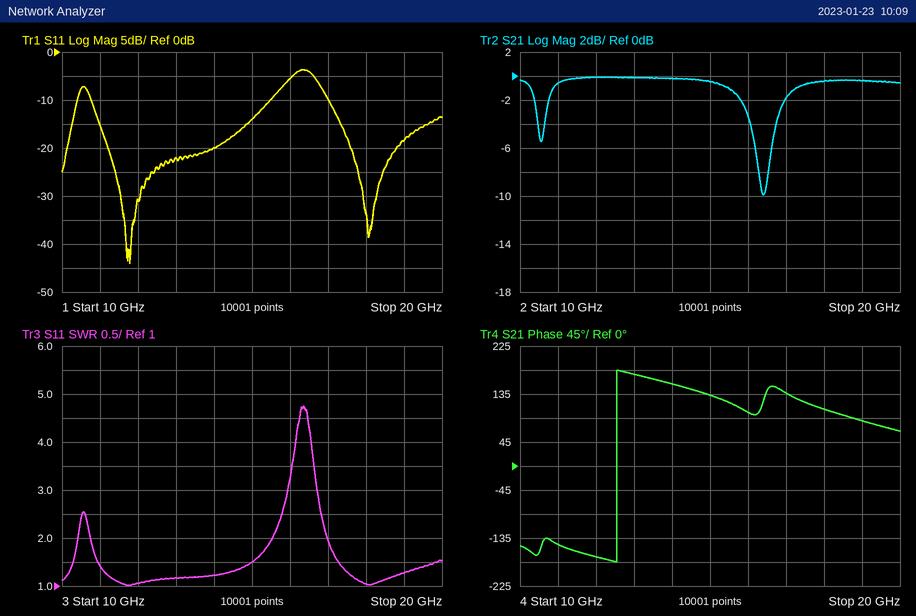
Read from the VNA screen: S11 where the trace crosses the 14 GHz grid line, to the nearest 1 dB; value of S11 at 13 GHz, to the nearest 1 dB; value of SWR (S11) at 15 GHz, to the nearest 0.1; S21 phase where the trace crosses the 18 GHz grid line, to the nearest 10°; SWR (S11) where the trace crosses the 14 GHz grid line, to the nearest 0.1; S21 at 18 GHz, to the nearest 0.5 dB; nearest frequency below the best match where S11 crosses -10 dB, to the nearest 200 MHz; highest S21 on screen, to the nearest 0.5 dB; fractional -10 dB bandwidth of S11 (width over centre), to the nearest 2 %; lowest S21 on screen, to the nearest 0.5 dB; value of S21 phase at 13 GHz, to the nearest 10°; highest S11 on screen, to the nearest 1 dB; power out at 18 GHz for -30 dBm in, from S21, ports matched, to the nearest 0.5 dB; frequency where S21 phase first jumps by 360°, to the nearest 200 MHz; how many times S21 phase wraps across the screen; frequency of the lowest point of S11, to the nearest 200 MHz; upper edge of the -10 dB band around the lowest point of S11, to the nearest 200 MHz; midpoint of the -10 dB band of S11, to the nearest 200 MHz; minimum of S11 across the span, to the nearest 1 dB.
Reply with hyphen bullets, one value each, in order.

- -20 dB
- -22 dB
- 1.5
- 110°
- 1.2
- -0.5 dB
- 10.8 GHz
- 0.0 dB
- 36 %
- -10.0 dB
- 170°
- -4 dB
- -30.5 dBm
- 12.6 GHz
- 1
- 11.8 GHz
- 15.4 GHz
- 13.2 GHz
- -44 dB
